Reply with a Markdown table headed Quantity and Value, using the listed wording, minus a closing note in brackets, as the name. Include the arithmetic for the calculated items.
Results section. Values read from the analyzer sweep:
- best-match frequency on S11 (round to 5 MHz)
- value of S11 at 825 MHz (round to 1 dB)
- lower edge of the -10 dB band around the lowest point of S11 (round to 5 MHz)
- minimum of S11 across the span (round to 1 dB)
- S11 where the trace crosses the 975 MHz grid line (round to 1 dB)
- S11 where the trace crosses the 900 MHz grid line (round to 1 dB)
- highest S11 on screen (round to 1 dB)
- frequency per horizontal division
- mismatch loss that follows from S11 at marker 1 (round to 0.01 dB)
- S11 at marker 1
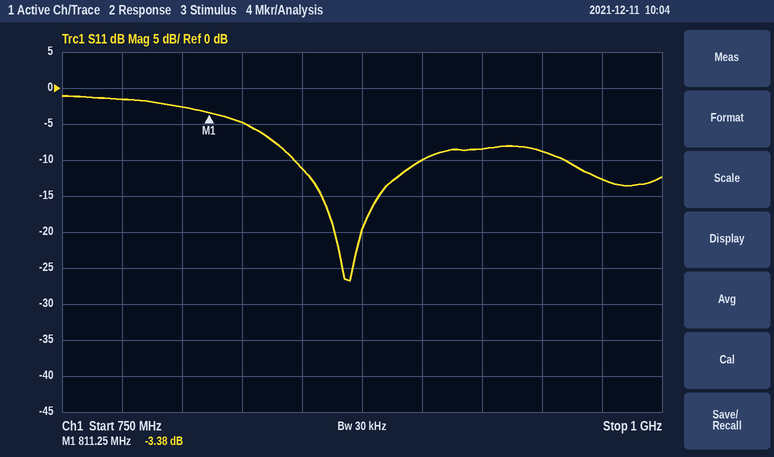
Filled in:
| Quantity | Value |
|---|---|
| best-match frequency on S11 | 870 MHz |
| value of S11 at 825 MHz | -5 dB |
| lower edge of the -10 dB band around the lowest point of S11 | 845 MHz |
| minimum of S11 across the span | -27 dB |
| S11 where the trace crosses the 975 MHz grid line | -13 dB |
| S11 where the trace crosses the 900 MHz grid line | -10 dB |
| highest S11 on screen | -1 dB |
| frequency per horizontal division | 25 MHz |
| mismatch loss that follows from S11 at marker 1 | −10 log10(1 − 10^(-3.38/10)) ≈ 2.67 dB |
| S11 at marker 1 | -3.38 dB |
